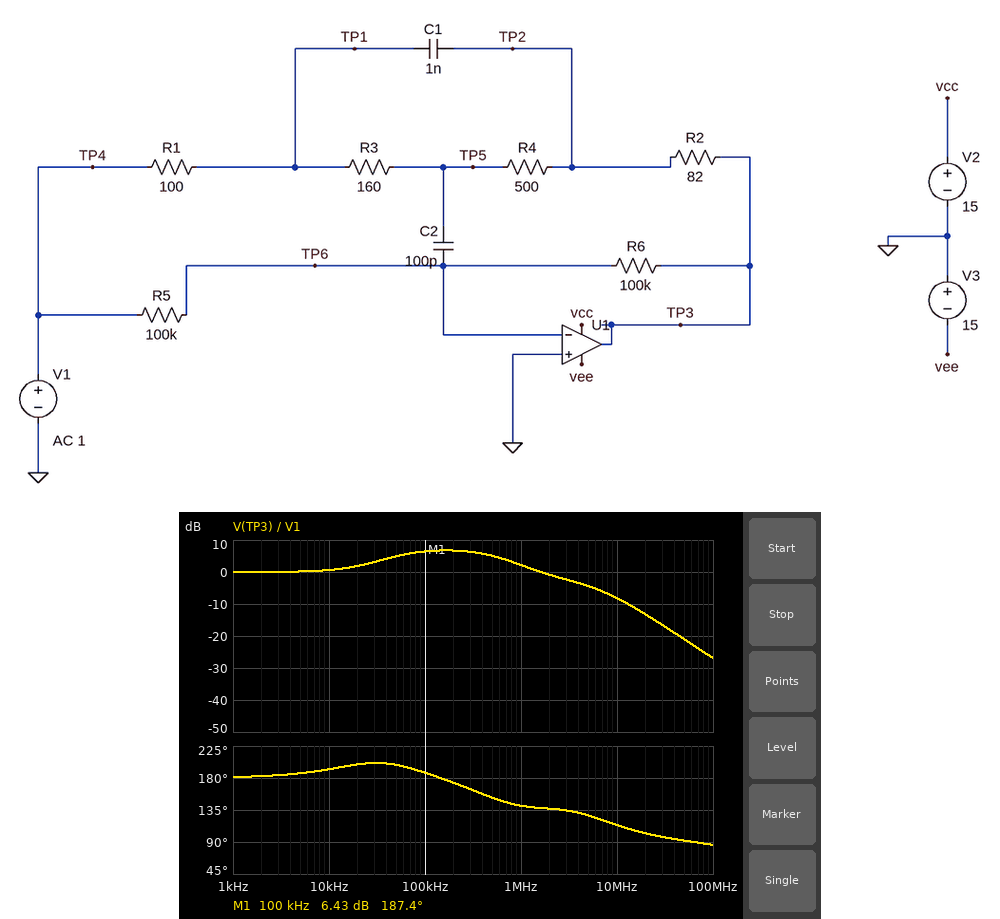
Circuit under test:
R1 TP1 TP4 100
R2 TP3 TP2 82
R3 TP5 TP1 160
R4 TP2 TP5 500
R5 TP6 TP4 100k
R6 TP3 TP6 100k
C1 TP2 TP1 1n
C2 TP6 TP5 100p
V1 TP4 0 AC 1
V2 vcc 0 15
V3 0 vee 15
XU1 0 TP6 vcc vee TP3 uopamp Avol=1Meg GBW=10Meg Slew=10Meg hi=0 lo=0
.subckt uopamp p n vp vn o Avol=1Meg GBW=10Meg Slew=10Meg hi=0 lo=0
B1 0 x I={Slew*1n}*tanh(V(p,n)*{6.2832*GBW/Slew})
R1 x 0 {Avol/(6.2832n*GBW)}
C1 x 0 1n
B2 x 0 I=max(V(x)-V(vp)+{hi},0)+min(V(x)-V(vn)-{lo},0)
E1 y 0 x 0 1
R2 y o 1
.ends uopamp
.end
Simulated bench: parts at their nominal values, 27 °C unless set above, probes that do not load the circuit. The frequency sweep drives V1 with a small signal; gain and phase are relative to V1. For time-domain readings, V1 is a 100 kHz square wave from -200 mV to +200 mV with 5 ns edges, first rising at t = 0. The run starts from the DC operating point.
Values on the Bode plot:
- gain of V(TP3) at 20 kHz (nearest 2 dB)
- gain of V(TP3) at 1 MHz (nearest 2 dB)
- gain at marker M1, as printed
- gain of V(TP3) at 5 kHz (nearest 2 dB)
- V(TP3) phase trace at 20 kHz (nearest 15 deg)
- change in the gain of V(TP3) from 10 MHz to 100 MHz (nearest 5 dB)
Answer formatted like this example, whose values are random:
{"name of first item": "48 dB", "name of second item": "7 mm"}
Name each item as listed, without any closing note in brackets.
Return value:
{"gain of V(TP3) at 20 kHz": "2 dB", "gain of V(TP3) at 1 MHz": "2 dB", "gain at marker M1, as printed": "6.43 dB", "gain of V(TP3) at 5 kHz": "0 dB", "V(TP3) phase trace at 20 kHz": "195 deg", "change in the gain of V(TP3) from 10 MHz to 100 MHz": "-20 dB"}
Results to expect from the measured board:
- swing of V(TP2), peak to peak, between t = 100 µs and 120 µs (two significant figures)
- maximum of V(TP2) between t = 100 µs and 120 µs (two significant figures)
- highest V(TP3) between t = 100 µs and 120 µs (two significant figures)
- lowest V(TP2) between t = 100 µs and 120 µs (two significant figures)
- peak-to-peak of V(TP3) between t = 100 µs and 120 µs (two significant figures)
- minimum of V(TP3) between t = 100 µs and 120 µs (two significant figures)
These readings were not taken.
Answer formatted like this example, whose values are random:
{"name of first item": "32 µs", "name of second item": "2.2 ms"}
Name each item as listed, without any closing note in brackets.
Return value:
{"swing of V(TP2), peak to peak, between t = 100 µs and 120 µs": "910 mV", "maximum of V(TP2) between t = 100 µs and 120 µs": "460 mV", "highest V(TP3) between t = 100 µs and 120 µs": "530 mV", "lowest V(TP2) between t = 100 µs and 120 µs": "-460 mV", "peak-to-peak of V(TP3) between t = 100 µs and 120 µs": "1.1 V", "minimum of V(TP3) between t = 100 µs and 120 µs": "-530 mV"}
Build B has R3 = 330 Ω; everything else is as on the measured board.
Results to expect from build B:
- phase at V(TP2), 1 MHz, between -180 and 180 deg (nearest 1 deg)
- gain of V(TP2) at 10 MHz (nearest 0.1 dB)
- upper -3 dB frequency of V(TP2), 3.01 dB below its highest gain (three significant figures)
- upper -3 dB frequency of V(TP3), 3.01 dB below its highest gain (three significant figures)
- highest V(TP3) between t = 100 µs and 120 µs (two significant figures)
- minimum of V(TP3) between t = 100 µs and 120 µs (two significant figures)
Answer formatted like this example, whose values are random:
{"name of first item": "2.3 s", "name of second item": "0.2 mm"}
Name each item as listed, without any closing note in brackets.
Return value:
{"phase at V(TP2), 1 MHz, between -180 and 180 deg": "118 deg", "gain of V(TP2) at 10 MHz": "-7.2 dB", "upper -3 dB frequency of V(TP2), 3.01 dB below its highest gain": "914 kHz", "upper -3 dB frequency of V(TP3), 3.01 dB below its highest gain": "1.31 MHz", "highest V(TP3) between t = 100 µs and 120 µs": "290 mV", "minimum of V(TP3) between t = 100 µs and 120 µs": "-290 mV"}
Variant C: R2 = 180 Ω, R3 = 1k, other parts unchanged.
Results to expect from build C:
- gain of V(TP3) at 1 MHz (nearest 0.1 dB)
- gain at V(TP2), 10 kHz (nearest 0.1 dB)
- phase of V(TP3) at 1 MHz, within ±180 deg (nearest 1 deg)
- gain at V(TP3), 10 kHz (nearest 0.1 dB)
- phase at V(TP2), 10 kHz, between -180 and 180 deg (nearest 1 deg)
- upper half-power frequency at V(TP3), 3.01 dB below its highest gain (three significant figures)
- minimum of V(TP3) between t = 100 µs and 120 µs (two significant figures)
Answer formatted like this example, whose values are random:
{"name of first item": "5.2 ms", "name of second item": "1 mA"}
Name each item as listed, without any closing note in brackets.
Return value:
{"gain of V(TP3) at 1 MHz": "2.2 dB", "gain at V(TP2), 10 kHz": "-2.4 dB", "phase of V(TP3) at 1 MHz, within ±180 deg": "-165 deg", "gain at V(TP3), 10 kHz": "-0.4 dB", "phase at V(TP2), 10 kHz, between -180 and 180 deg": "170 deg", "upper half-power frequency at V(TP3), 3.01 dB below its highest gain": "4.97 MHz", "minimum of V(TP3) between t = 100 µs and 120 µs": "-360 mV"}
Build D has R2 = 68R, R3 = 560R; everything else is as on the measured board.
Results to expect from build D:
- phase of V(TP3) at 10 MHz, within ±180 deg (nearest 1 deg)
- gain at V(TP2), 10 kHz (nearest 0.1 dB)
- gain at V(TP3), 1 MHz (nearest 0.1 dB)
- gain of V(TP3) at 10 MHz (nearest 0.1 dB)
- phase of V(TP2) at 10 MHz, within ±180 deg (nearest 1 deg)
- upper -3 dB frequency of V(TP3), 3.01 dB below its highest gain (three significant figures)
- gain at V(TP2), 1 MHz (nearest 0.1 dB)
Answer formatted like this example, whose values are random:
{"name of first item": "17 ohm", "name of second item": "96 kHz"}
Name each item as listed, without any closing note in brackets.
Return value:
{"phase of V(TP3) at 10 MHz, within ±180 deg": "119 deg", "gain at V(TP2), 10 kHz": "-1.1 dB", "gain at V(TP3), 1 MHz": "-2.4 dB", "gain of V(TP3) at 10 MHz": "-9.2 dB", "phase of V(TP2) at 10 MHz, within ±180 deg": "36 deg", "upper -3 dB frequency of V(TP3), 3.01 dB below its highest gain": "1.55 MHz", "gain at V(TP2), 1 MHz": "-4.8 dB"}
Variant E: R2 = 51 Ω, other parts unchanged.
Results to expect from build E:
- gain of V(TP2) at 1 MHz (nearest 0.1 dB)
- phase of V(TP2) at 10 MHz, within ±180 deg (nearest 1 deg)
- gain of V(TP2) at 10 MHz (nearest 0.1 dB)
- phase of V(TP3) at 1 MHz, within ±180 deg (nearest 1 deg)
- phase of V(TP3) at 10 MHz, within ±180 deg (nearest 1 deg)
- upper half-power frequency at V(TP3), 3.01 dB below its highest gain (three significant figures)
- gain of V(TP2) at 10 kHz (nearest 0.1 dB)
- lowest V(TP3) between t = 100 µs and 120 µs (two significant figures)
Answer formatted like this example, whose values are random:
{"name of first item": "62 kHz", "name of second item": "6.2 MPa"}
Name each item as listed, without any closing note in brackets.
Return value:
{"gain of V(TP2) at 1 MHz": "-0.1 dB", "phase of V(TP2) at 10 MHz, within ±180 deg": "38 deg", "gain of V(TP2) at 10 MHz": "-9.4 dB", "phase of V(TP3) at 1 MHz, within ±180 deg": "133 deg", "phase of V(TP3) at 10 MHz, within ±180 deg": "114 deg", "upper half-power frequency at V(TP3), 3.01 dB below its highest gain": "650 kHz", "gain of V(TP2) at 10 kHz": "-0.5 dB", "lowest V(TP3) between t = 100 µs and 120 µs": "-500 mV"}
